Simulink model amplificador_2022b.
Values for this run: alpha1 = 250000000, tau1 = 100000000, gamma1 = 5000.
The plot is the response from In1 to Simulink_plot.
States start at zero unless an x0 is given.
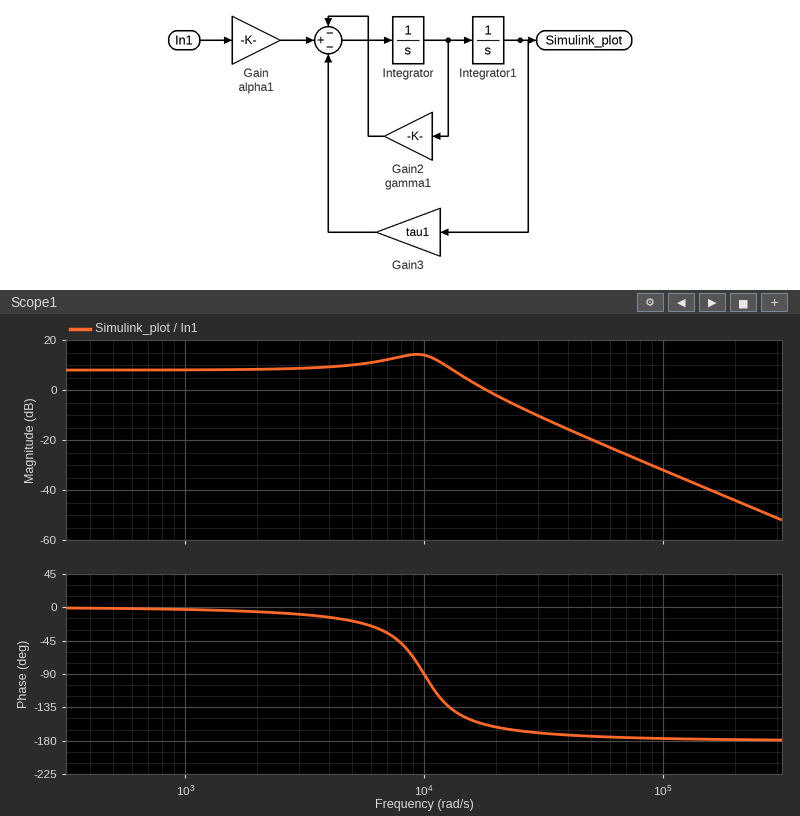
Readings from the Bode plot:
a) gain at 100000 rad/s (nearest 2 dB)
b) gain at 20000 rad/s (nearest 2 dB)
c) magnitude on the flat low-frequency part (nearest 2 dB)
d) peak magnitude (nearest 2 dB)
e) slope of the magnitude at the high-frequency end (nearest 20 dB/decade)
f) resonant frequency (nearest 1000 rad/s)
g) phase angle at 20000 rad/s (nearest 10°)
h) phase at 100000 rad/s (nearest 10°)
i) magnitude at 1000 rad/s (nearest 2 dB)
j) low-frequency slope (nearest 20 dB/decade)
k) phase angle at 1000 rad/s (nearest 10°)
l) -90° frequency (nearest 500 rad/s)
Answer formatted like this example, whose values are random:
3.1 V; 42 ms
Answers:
-32 dB; -2 dB; 8 dB; 14 dB; -40 dB/decade; 9000 rad/s; -160°; -180°; 8 dB; 0 dB/decade; 0°; 10000 rad/s
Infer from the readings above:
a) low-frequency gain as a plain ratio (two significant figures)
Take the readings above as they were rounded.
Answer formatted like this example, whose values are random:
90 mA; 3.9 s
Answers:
2.5
